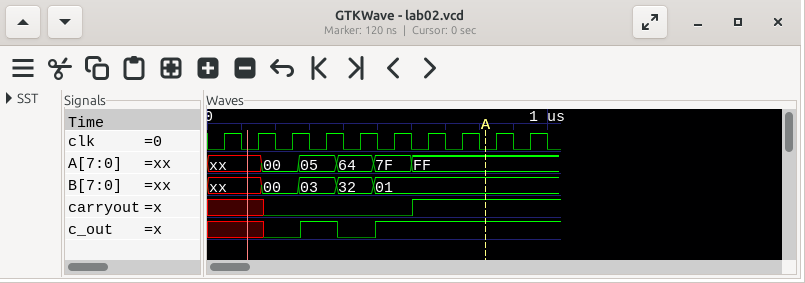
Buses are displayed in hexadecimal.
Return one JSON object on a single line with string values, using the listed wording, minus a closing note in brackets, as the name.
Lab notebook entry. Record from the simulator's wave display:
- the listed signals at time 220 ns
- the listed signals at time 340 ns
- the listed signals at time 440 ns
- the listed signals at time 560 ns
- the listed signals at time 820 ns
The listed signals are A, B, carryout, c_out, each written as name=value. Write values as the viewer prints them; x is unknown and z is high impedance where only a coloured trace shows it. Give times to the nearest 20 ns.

{"the listed signals at time 220 ns": "A=00, B=00, carryout=0, c_out=0", "the listed signals at time 340 ns": "A=05, B=03, carryout=0, c_out=1", "the listed signals at time 440 ns": "A=64, B=32, carryout=0, c_out=0", "the listed signals at time 560 ns": "A=7F, B=01, carryout=0, c_out=1", "the listed signals at time 820 ns": "A=FF, B=01, carryout=1, c_out=1"}
